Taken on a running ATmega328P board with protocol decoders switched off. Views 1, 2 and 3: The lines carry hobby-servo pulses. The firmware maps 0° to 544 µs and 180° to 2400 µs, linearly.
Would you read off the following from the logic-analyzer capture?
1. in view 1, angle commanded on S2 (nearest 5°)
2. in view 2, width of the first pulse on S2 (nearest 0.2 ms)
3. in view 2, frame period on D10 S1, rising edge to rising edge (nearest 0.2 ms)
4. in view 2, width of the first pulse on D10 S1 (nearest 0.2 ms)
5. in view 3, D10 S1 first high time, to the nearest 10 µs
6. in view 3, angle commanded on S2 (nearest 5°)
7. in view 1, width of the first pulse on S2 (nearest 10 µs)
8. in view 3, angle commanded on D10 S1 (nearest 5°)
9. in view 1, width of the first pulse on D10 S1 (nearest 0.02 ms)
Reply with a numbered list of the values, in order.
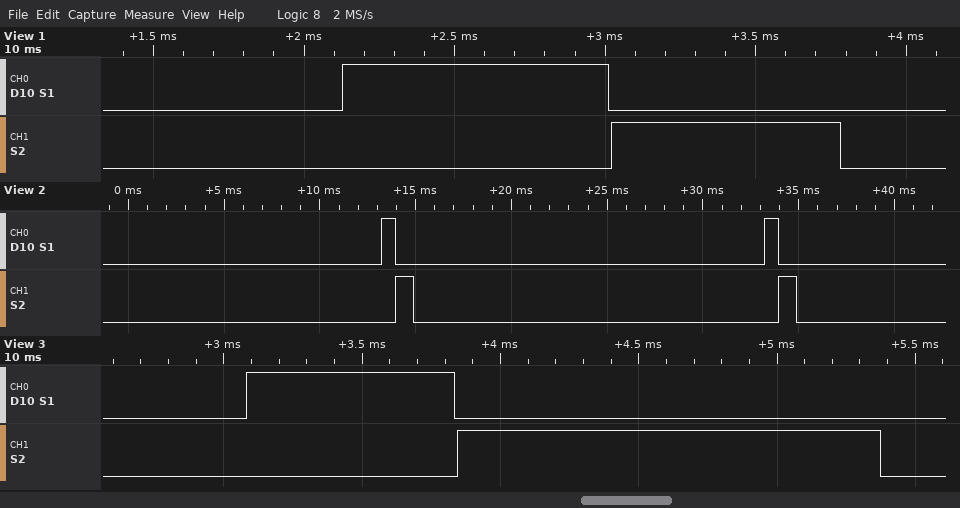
1. 20°
2. 1.0 ms
3. 20.0 ms
4. 0.8 ms
5. 750 µs
6. 95°
7. 760 µs
8. 20°
9. 0.88 ms
